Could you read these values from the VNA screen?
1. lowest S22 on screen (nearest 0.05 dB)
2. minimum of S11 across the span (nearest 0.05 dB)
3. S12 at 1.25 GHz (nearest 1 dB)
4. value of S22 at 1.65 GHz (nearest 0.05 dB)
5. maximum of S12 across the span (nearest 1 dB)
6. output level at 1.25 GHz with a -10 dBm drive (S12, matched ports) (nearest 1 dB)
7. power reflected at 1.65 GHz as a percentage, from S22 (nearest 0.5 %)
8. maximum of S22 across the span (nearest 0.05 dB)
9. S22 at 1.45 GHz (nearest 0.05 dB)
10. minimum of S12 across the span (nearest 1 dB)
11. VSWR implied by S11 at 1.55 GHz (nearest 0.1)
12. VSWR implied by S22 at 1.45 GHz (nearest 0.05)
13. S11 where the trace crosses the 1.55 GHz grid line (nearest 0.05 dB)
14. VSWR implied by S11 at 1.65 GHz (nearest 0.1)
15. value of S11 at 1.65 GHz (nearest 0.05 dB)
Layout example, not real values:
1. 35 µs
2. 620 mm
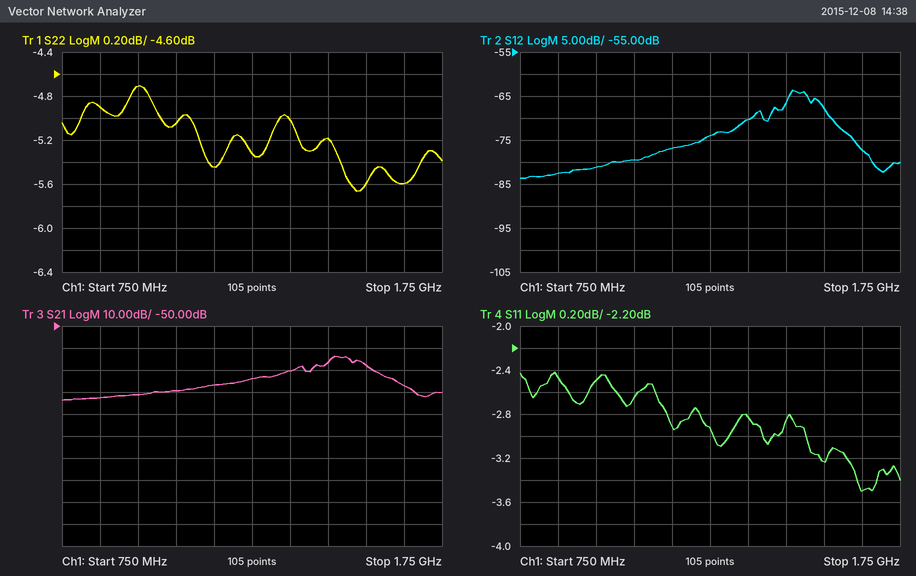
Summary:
1. -5.65 dB
2. -3.50 dB
3. -74 dB
4. -5.60 dB
5. -64 dB
6. -84 dBm
7. 27.5 %
8. -4.70 dB
9. -5.20 dB
10. -84 dB
11. 5.4
12. 3.45
13. -3.25 dB
14. 5.0
15. -3.50 dB
